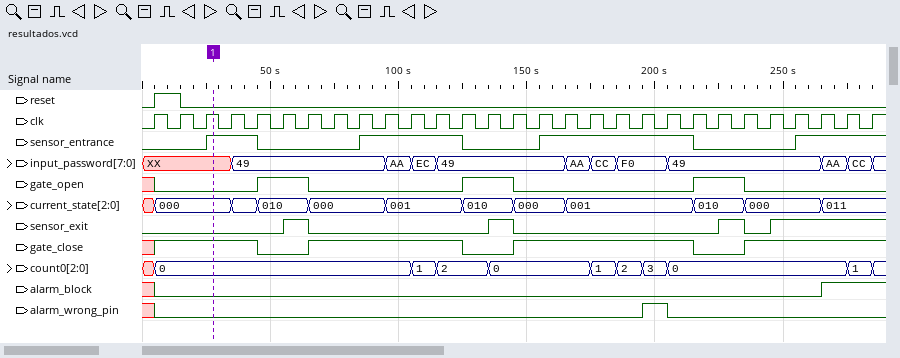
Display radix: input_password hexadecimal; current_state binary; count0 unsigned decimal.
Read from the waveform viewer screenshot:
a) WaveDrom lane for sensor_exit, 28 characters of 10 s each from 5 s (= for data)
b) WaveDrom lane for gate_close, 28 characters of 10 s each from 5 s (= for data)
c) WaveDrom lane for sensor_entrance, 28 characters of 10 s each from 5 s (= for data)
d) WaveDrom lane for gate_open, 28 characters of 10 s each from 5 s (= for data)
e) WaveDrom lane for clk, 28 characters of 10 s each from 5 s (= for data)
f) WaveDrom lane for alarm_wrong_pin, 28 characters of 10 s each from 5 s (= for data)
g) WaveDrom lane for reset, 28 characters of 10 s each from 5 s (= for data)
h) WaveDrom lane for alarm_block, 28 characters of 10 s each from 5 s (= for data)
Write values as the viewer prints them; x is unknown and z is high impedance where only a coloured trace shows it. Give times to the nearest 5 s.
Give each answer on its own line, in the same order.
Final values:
{name: 'sensor_exit', wave: '0....10......10.......101...'}
{name: 'gate_close', wave: '1...0.1.....0.1......0.1....'}
{name: 'sensor_entrance', wave: '0.1.0...1...0..1.....0...1..'}
{name: 'gate_open', wave: '0...1.0.....1.0......1.0....'}
{name: 'clk', wave: 'p...........................'}
{name: 'alarm_wrong_pin', wave: '0..................10.......'}
{name: 'reset', wave: '10..........................'}
{name: 'alarm_block', wave: '0.........................1.'}
